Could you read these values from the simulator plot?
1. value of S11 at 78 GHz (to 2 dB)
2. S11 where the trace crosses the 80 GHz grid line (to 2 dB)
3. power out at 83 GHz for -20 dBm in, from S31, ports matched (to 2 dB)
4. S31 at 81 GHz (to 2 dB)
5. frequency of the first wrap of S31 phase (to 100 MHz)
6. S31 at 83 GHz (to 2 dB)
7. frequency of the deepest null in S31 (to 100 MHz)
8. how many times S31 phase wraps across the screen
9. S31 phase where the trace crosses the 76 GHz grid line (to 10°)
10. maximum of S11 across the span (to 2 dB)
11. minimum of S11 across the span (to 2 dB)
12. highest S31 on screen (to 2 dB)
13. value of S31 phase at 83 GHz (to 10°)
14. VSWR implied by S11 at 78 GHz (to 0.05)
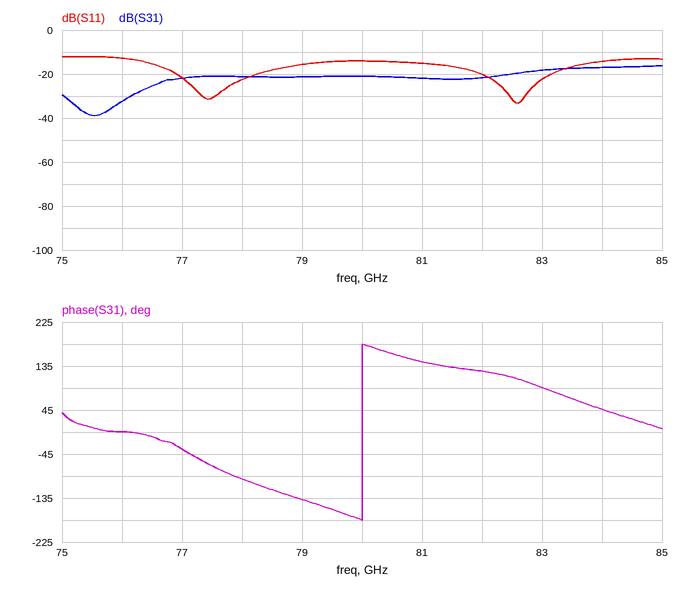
-22 dB
-14 dB
-38 dBm
-22 dB
80.0 GHz
-18 dB
75.5 GHz
1
0°
-12 dB
-34 dB
-16 dB
90°
1.15
